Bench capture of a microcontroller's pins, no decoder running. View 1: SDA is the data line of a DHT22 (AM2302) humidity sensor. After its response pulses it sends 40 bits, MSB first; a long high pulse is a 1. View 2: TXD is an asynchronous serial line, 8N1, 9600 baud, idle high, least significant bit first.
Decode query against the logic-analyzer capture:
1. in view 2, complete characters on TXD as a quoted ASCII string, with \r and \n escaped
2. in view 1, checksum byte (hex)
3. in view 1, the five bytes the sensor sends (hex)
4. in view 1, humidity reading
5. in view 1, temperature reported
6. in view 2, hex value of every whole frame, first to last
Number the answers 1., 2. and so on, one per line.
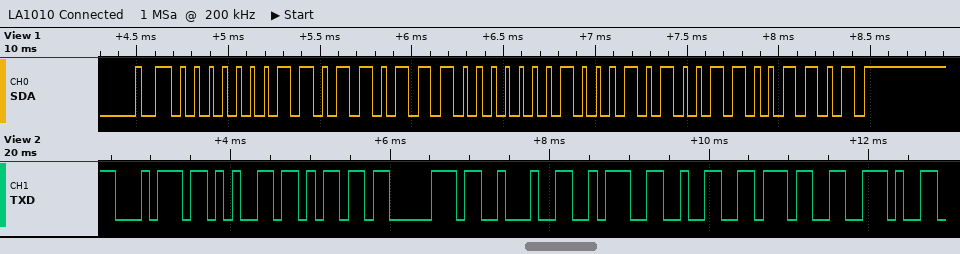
1. "temp\":27."
2. 0xCD
3. 01 B7 01 14 CD
4. 43.9 %
5. 27.6 °C
6. 0x74 0x65 0x6D 0x70 0x22 0x3A 0x32 0x37 0x2E
